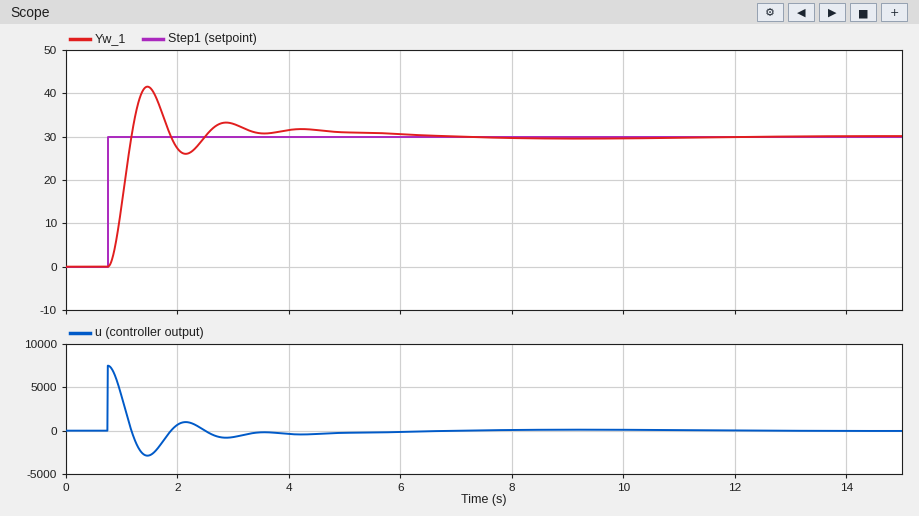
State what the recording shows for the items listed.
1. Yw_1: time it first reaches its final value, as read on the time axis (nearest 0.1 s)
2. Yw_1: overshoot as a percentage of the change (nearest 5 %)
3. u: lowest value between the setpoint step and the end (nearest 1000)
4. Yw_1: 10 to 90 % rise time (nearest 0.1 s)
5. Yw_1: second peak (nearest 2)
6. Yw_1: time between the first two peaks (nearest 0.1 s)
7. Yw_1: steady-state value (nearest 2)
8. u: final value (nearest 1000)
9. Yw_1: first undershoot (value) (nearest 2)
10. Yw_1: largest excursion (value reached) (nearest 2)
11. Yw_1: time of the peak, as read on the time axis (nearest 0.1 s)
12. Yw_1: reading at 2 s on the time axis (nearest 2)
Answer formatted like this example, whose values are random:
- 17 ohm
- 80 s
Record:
- 1.2 s
- 40 %
- -3000
- 0.3 s
- 34
- 1.4 s
- 30
- 0
- 26
- 42
- 1.5 s
- 28
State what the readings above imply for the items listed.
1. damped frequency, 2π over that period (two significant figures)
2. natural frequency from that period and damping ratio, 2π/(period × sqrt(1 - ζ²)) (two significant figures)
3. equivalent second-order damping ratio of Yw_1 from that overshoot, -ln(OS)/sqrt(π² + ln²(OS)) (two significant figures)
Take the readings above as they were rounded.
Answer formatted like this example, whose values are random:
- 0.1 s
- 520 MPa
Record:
- 4.5 rad/s
- 4.7 rad/s
- 0.28
